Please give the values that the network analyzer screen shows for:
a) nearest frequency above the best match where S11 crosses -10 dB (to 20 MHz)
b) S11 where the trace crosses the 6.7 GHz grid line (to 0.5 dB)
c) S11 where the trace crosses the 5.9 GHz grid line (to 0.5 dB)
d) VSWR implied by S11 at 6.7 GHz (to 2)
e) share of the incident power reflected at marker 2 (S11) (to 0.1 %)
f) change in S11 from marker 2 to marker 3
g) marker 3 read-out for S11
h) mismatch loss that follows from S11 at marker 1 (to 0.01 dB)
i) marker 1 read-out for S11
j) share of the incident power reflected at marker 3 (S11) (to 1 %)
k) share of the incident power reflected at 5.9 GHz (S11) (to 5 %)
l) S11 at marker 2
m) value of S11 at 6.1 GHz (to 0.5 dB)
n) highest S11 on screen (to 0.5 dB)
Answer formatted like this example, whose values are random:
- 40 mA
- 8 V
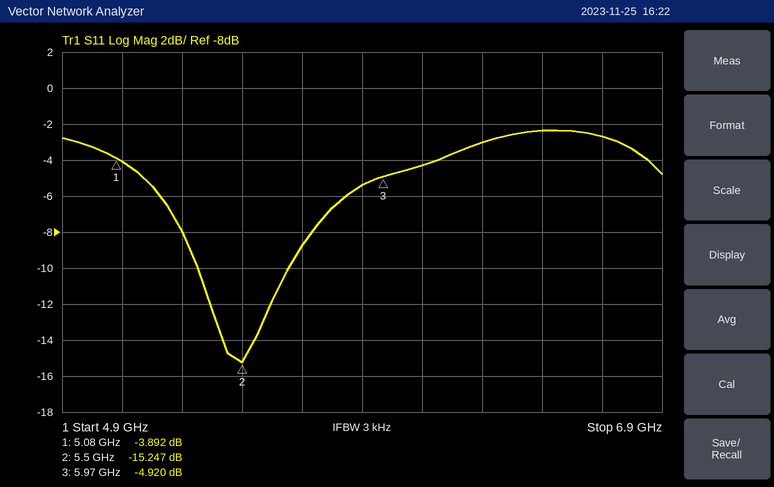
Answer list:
- 5.66 GHz
- -2.5 dB
- -5.5 dB
- 6
- 3.0 %
- 10.327 dB
- -4.920 dB
- 2.28 dB
- -3.892 dB
- 32 %
- 30 %
- -15.247 dB
- -4.5 dB
- -2.5 dB
